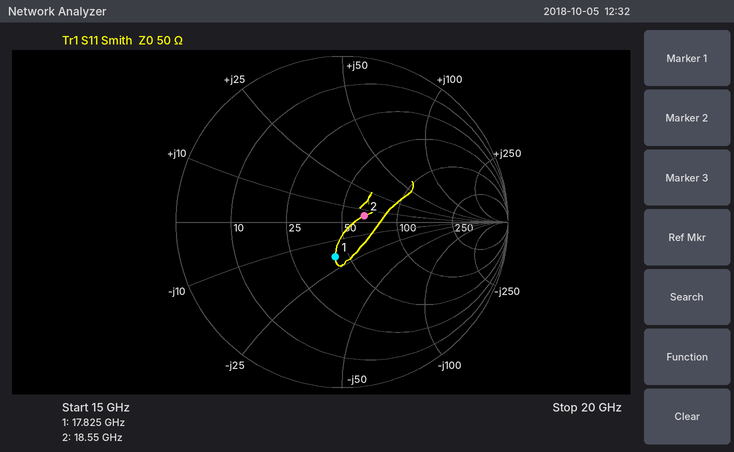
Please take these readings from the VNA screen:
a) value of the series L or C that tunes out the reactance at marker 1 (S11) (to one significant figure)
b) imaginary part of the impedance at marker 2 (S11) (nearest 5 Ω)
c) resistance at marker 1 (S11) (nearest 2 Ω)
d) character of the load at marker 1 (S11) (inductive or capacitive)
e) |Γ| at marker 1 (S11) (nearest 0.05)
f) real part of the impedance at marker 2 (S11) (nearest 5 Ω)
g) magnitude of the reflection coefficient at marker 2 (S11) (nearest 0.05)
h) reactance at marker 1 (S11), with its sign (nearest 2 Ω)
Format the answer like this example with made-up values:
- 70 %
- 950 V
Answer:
- 200 pH
- +5 Ω
- 42 Ω
- capacitive
- 0.20
- 65 Ω
- 0.15
- -18 Ω
